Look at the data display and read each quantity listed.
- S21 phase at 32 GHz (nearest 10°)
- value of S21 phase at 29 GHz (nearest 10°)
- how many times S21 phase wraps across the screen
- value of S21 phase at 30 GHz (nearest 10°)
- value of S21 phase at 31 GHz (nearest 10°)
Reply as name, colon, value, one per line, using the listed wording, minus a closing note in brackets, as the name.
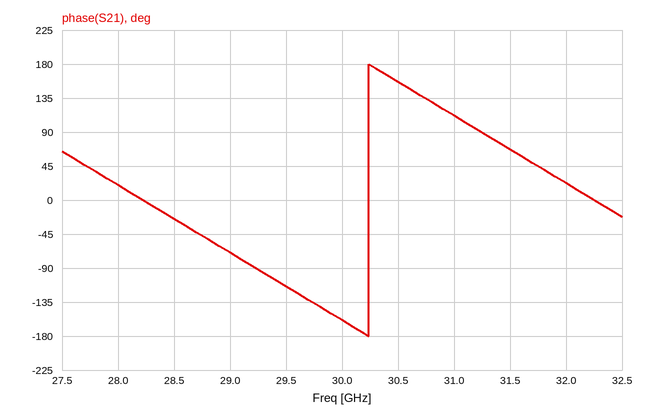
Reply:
S21 phase at 32 GHz: 20°
value of S21 phase at 29 GHz: -70°
how many times S21 phase wraps across the screen: 1
value of S21 phase at 30 GHz: -160°
value of S21 phase at 31 GHz: 110°
